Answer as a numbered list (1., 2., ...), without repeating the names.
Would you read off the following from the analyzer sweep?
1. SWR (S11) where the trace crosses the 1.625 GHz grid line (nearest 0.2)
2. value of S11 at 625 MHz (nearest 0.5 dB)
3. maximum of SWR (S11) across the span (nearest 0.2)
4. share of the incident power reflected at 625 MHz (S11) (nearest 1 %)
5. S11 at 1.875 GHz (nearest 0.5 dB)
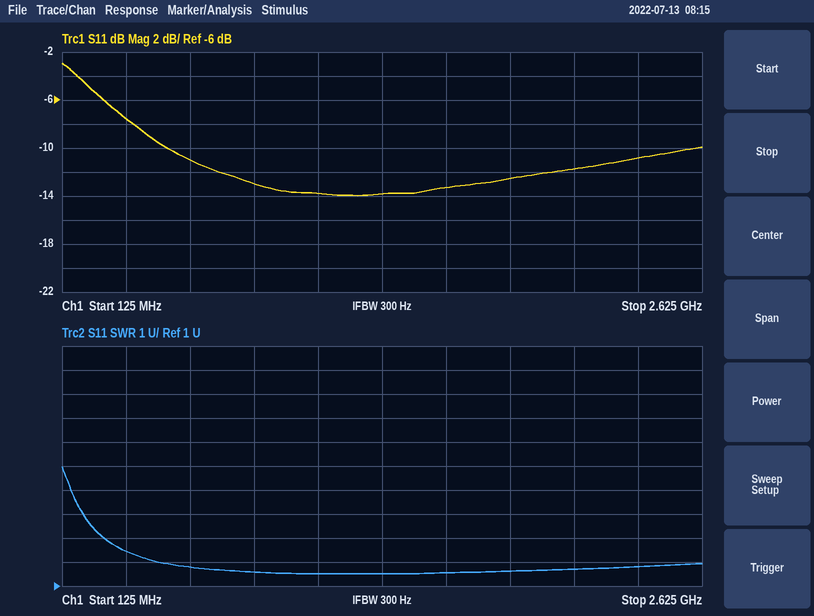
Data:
1. 1.6
2. -11.0 dB
3. 6.0
4. 8 %
5. -12.5 dB
